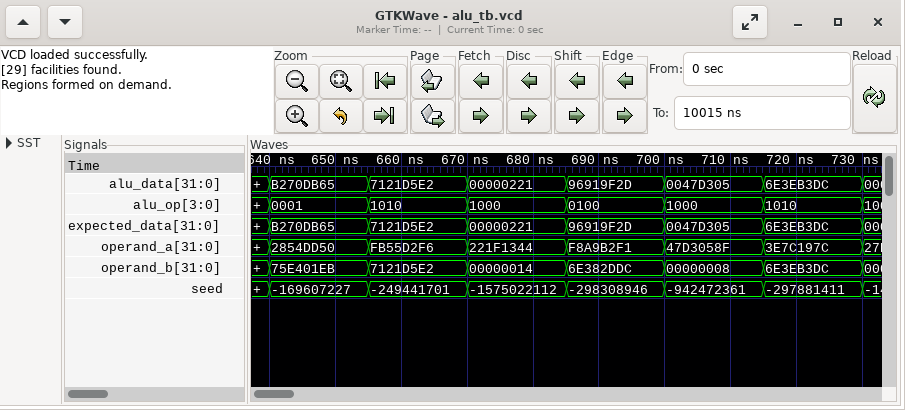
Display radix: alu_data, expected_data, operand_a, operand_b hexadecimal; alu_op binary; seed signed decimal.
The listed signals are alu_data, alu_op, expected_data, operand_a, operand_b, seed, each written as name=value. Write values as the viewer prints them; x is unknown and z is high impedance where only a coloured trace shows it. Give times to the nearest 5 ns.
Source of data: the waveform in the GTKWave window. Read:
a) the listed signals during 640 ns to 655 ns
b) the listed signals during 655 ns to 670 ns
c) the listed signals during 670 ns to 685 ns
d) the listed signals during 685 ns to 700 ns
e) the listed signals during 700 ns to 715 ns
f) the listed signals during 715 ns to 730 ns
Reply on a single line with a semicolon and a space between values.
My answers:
alu_data=B270DB65, alu_op=0001, expected_data=B270DB65, operand_a=2854DD50, operand_b=75E401EB, seed=-169607227; alu_data=7121D5E2, alu_op=1010, expected_data=7121D5E2, operand_a=FB55D2F6, operand_b=7121D5E2, seed=-249441701; alu_data=00000221, alu_op=1000, expected_data=00000221, operand_a=221F1344, operand_b=00000014, seed=-1575022112; alu_data=96919F2D, alu_op=0100, expected_data=96919F2D, operand_a=F8A9B2F1, operand_b=6E382DDC, seed=-298308946; alu_data=0047D305, alu_op=1000, expected_data=0047D305, operand_a=47D3058F, operand_b=00000008, seed=-942472361; alu_data=6E3EB3DC, alu_op=1010, expected_data=6E3EB3DC, operand_a=3E7C197C, operand_b=6E3EB3DC, seed=-297881411
